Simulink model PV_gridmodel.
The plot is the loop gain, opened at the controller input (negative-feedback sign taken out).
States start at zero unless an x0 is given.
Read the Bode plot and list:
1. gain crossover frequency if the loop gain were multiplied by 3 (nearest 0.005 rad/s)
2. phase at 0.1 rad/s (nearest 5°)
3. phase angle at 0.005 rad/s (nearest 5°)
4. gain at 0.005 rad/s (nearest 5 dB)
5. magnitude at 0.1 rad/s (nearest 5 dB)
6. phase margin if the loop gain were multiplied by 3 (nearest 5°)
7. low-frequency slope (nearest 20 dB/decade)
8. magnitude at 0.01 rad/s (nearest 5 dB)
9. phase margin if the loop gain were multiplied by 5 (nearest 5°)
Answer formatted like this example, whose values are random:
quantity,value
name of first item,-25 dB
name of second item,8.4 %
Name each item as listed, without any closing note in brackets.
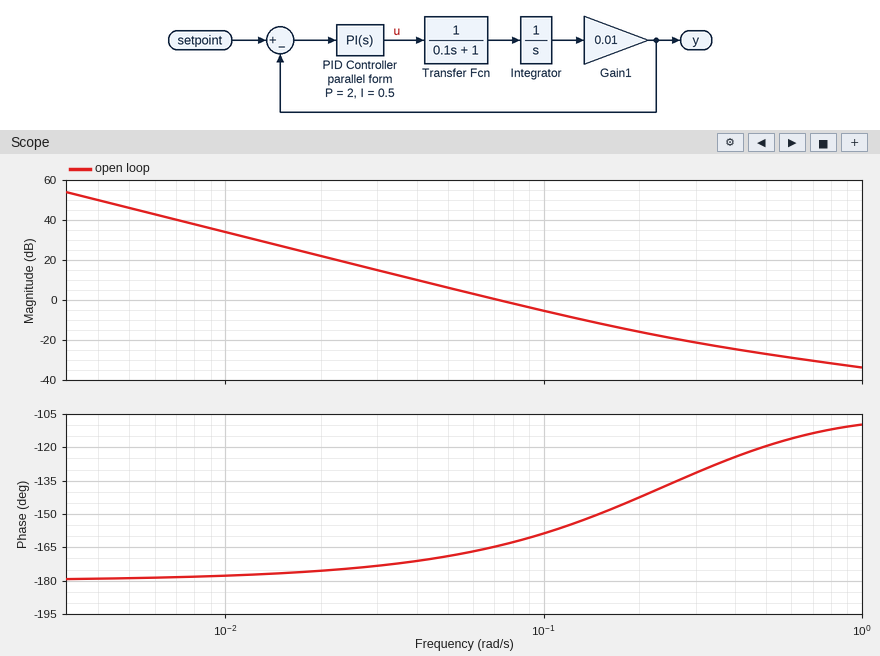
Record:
quantity,value
gain crossover frequency if the loop gain were multiplied by 3,0.130 rad/s
phase at 0.1 rad/s,-160°
phase angle at 0.005 rad/s,-180°
gain at 0.005 rad/s,45 dB
magnitude at 0.1 rad/s,-5 dB
phase margin if the loop gain were multiplied by 3,25°
low-frequency slope,-40 dB/decade
magnitude at 0.01 rad/s,35 dB
phase margin if the loop gain were multiplied by 5,35°
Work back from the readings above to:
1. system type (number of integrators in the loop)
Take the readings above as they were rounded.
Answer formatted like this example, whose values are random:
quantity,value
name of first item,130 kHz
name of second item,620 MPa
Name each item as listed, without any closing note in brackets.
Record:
quantity,value
system type,2
